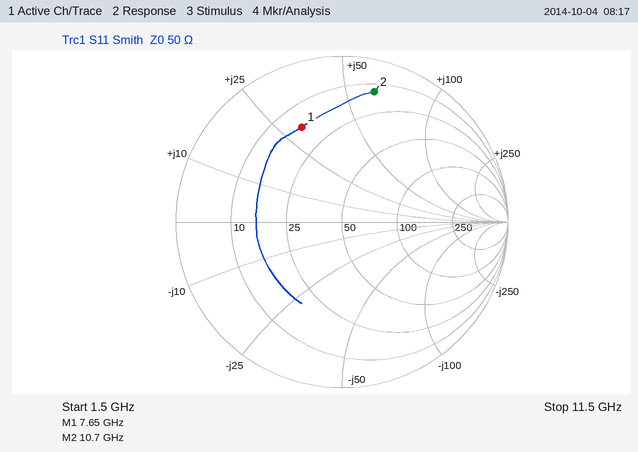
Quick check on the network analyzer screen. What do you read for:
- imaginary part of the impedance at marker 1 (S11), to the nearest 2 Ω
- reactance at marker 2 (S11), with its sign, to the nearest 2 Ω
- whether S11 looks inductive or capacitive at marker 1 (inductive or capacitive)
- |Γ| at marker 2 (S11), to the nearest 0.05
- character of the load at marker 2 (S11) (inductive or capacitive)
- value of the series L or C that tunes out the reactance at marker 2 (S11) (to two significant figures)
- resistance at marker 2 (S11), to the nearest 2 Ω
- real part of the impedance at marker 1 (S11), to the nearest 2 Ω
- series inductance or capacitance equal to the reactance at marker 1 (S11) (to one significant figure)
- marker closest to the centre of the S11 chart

+30 Ω
+62 Ω
inductive
0.80
inductive
240 fF
14 Ω
16 Ω
600 pH
marker 1
